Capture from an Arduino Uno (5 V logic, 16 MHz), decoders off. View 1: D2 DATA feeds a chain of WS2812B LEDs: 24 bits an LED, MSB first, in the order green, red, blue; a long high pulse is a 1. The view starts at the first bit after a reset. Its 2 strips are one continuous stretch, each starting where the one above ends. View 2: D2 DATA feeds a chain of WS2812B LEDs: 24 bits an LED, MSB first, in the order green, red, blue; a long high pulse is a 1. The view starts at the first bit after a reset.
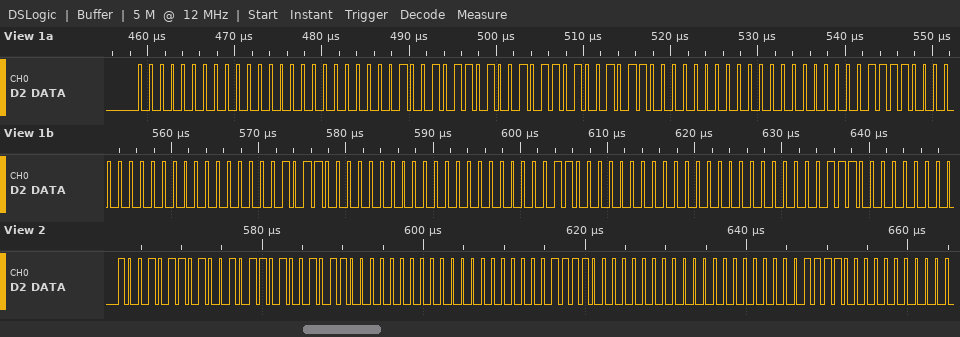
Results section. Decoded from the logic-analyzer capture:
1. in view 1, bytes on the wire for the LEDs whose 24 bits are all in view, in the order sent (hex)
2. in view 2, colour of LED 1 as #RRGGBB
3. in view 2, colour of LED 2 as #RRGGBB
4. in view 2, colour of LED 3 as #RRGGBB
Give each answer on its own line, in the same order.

00 00 00 96 96 96 00 00 1E 00 00 16 00 00 0C 00 00 07
#969696
#00001E
#00000F
